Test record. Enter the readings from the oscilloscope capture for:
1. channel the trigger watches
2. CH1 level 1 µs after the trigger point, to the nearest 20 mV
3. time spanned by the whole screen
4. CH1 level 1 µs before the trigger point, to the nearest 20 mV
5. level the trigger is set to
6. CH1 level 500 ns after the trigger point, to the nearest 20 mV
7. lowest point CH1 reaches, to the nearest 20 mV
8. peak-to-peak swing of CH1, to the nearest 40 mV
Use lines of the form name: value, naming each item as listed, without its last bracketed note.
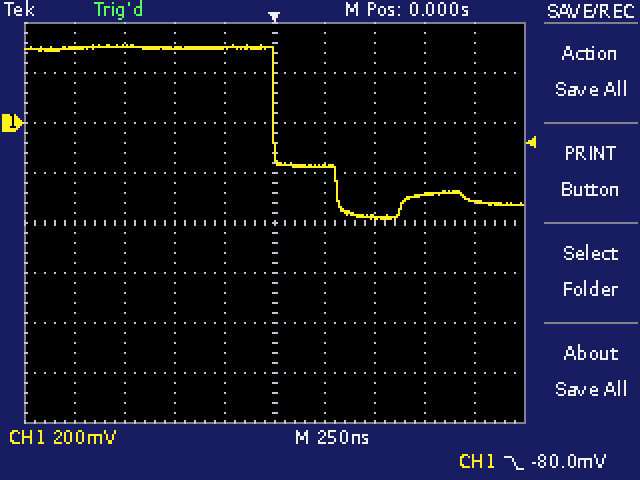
channel the trigger watches: CH1
CH1 level 1 µs after the trigger point, to the nearest 20 mV: -320 mV
time spanned by the whole screen: 2.5 µs
CH1 level 1 µs before the trigger point, to the nearest 20 mV: 300 mV
level the trigger is set to: -80.0 mV
CH1 level 500 ns after the trigger point, to the nearest 20 mV: -380 mV
lowest point CH1 reaches, to the nearest 20 mV: -380 mV
peak-to-peak swing of CH1, to the nearest 40 mV: 680 mV
